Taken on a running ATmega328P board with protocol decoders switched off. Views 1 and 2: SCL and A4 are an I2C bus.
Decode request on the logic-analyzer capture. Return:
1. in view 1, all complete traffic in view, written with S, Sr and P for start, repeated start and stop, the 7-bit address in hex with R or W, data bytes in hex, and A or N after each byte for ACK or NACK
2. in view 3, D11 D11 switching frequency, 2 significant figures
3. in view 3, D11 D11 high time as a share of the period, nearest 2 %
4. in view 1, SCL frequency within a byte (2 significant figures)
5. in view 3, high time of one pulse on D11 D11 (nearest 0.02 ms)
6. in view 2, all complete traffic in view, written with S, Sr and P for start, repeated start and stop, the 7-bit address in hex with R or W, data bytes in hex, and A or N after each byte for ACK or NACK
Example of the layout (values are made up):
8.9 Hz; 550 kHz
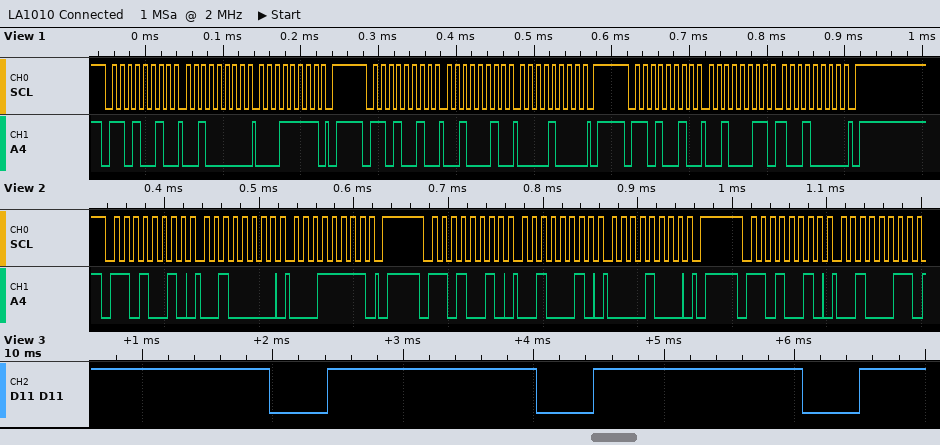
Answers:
S 69W A 20 A 1F A P S 69W A 22 A 08 A P S 69W A 23 A 90 A P; 490 Hz; 78 %; 100 kHz; 1.60 ms; S 69W A 20 A 1F A P S 69W A 22 A 08 A P S 69W A 23 A
